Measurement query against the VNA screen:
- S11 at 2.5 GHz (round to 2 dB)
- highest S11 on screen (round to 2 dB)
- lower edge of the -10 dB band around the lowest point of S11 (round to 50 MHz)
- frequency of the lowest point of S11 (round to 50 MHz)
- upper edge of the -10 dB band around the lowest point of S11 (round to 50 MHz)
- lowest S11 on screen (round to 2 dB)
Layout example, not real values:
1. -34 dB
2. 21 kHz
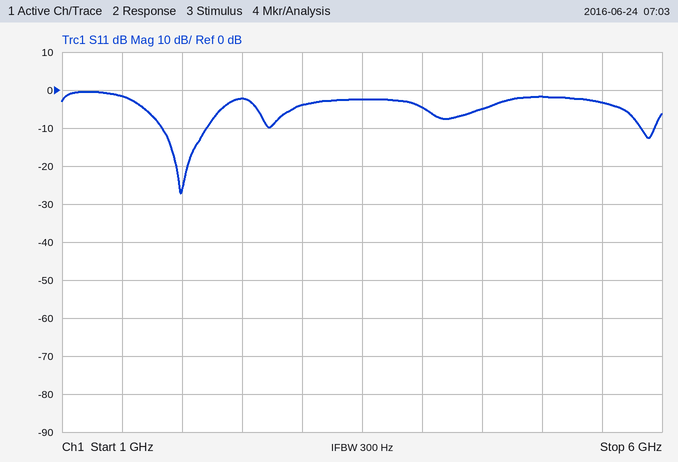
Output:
1. -2 dB
2. 0 dB
3. 1.85 GHz
4. 2.00 GHz
5. 2.20 GHz
6. -28 dB
